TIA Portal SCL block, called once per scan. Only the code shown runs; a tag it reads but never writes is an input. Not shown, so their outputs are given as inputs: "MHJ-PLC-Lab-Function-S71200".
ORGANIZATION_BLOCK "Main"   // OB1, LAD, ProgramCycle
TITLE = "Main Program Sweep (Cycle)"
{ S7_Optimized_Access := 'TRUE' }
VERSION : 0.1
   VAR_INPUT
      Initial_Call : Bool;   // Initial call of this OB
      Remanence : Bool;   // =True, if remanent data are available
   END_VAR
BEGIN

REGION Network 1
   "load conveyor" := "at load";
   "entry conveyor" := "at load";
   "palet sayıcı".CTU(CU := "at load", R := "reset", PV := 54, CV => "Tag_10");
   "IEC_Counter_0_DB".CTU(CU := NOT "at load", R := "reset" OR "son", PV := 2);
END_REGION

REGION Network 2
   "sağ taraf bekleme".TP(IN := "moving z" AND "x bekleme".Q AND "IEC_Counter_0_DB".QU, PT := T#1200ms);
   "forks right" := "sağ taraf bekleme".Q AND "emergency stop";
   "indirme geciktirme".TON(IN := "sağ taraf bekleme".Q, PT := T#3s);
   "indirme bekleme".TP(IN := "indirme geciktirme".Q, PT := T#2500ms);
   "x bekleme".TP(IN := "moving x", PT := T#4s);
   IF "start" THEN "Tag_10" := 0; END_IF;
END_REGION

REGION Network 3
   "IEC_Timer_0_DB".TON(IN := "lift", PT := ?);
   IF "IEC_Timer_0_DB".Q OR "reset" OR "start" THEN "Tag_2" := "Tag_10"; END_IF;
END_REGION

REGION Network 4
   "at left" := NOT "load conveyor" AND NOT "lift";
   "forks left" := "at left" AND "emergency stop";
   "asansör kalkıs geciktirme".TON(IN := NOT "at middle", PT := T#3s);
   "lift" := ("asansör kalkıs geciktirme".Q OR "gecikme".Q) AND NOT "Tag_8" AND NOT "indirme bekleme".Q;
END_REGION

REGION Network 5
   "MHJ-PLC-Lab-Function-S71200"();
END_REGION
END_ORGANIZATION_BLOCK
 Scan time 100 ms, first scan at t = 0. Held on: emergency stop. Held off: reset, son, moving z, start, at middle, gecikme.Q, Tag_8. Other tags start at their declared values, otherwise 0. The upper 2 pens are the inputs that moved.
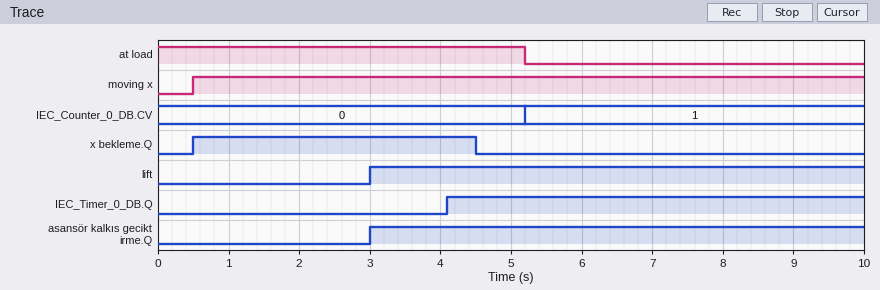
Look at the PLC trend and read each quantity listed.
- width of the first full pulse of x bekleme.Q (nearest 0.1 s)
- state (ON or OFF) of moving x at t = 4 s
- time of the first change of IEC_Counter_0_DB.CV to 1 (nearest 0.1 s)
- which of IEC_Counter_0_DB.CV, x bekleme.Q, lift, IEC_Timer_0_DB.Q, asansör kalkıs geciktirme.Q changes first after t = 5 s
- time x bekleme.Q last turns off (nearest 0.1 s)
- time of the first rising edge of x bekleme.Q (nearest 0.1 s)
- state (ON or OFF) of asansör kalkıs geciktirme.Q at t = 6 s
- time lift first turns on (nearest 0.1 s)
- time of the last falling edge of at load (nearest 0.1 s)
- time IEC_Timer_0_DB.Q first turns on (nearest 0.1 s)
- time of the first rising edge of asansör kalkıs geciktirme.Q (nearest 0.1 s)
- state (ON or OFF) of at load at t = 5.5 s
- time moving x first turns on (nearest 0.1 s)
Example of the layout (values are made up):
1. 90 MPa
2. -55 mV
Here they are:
1. 4.0 s
2. ON
3. 5.2 s
4. IEC_Counter_0_DB.CV
5. 4.5 s
6. 0.5 s
7. ON
8. 3.0 s
9. 5.2 s
10. 4.1 s
11. 3.0 s
12. OFF
13. 0.5 s
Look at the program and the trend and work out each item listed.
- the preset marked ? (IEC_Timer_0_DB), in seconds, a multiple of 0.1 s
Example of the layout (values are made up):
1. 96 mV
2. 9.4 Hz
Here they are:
1. 1.0 s
